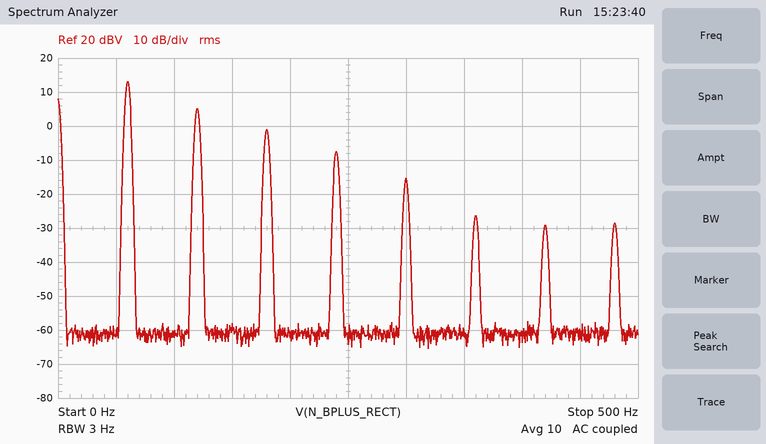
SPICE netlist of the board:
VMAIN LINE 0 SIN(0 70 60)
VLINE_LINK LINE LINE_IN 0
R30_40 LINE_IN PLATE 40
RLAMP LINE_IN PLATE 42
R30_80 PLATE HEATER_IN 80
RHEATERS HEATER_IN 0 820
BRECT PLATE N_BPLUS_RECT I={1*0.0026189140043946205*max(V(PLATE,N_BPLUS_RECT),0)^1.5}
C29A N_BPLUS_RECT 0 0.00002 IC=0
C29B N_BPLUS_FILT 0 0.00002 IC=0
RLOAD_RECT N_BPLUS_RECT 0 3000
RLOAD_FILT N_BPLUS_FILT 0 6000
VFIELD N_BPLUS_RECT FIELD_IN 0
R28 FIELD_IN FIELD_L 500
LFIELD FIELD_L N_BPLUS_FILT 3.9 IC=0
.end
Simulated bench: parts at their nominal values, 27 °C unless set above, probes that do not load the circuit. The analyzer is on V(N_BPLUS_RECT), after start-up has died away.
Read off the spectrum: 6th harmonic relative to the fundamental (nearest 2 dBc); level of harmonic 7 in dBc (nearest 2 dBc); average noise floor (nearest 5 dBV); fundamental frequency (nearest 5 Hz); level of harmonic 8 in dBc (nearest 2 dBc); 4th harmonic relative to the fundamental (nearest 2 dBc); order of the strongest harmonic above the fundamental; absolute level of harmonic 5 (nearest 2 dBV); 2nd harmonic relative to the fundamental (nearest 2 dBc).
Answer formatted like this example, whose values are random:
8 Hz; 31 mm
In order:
-40 dBc; -42 dBc; -60 dBV; 60 Hz; -42 dBc; -20 dBc; 2; -16 dBV; -8 dBc
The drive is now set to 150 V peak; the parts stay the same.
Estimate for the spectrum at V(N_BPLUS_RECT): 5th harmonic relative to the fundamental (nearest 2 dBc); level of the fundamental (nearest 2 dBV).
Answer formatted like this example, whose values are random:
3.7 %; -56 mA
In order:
-26 dBc; 20 dBV
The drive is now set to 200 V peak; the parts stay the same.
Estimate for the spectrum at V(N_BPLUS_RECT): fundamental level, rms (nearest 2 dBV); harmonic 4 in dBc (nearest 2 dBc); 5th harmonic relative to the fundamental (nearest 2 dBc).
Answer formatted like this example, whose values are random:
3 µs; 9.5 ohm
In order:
22 dBV; -20 dBc; -26 dBc
